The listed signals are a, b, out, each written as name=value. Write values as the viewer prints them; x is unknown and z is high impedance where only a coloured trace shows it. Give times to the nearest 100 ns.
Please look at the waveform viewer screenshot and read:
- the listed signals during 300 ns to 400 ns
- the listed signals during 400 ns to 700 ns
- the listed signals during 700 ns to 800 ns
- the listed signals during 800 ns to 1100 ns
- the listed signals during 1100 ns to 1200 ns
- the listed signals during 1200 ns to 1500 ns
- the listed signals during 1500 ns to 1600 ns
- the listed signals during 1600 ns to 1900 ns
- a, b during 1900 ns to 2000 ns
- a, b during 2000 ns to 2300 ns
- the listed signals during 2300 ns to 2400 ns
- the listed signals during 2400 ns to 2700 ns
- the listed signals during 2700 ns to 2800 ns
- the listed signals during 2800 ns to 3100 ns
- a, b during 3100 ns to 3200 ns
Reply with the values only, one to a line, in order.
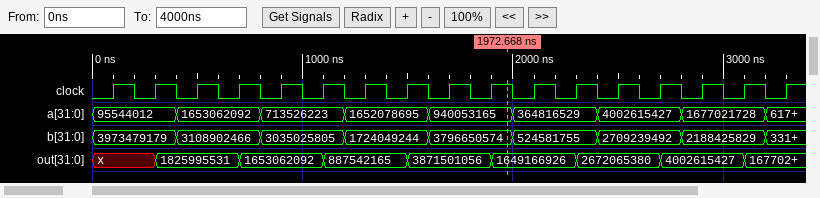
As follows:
a=95544012, b=3973479179, out=1825995531
a=1653062092, b=3108902466, out=1825995531
a=1653062092, b=3108902466, out=1653062092
a=713526223, b=3035025805, out=1653062092
a=713526223, b=3035025805, out=887542165
a=1652078695, b=1724049244, out=887542165
a=1652078695, b=1724049244, out=3871501056
a=940053165, b=3796650574, out=3871501056
a=940053165, b=3796650574
a=364816529, b=524581755
a=364816529, b=524581755, out=2672065380
a=4002615427, b=2709239492, out=2672065380
a=4002615427, b=2709239492, out=4002615427
a=1677021728, b=2188425829, out=4002615427
a=1677021728, b=2188425829
